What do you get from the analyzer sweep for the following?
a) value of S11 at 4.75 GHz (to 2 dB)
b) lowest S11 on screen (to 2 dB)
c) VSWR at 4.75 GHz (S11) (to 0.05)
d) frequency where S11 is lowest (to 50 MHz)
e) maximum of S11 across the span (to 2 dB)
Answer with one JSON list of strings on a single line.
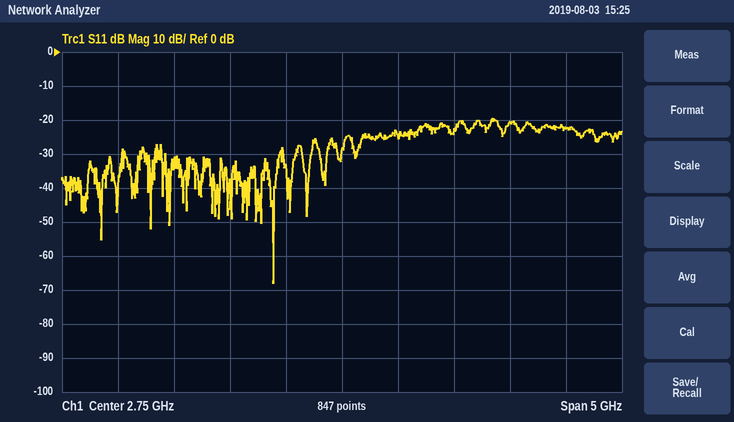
["-22 dB", "-68 dB", "1.15", "2.15 GHz", "-20 dB"]
